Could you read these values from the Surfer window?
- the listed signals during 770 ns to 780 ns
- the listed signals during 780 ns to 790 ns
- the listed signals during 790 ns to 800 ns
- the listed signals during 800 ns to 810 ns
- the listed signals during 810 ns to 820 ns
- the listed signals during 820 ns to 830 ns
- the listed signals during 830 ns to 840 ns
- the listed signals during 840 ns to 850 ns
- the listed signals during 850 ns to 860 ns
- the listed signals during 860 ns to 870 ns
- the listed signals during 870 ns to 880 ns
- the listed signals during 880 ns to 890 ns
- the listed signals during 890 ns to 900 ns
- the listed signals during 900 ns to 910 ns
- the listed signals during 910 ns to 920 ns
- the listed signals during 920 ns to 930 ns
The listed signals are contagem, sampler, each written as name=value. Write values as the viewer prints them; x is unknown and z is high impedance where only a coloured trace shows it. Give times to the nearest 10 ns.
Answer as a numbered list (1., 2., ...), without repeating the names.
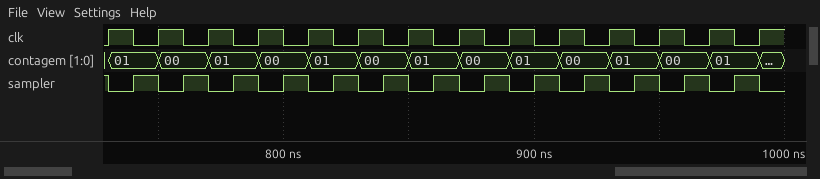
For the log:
1. contagem=01, sampler=0
2. contagem=01, sampler=1
3. contagem=00, sampler=0
4. contagem=00, sampler=1
5. contagem=01, sampler=0
6. contagem=01, sampler=1
7. contagem=00, sampler=0
8. contagem=00, sampler=1
9. contagem=01, sampler=0
10. contagem=01, sampler=1
11. contagem=00, sampler=0
12. contagem=00, sampler=1
13. contagem=01, sampler=0
14. contagem=01, sampler=1
15. contagem=00, sampler=0
16. contagem=00, sampler=1
